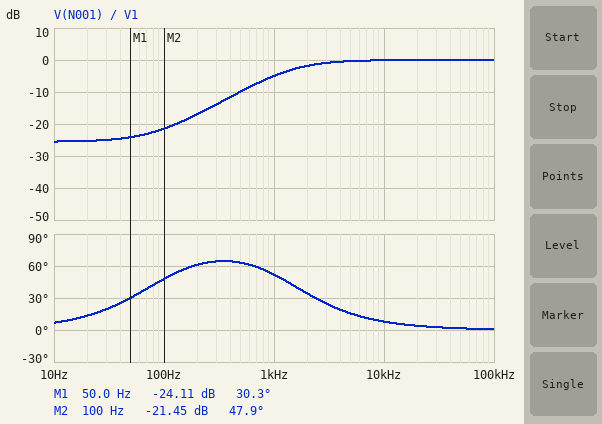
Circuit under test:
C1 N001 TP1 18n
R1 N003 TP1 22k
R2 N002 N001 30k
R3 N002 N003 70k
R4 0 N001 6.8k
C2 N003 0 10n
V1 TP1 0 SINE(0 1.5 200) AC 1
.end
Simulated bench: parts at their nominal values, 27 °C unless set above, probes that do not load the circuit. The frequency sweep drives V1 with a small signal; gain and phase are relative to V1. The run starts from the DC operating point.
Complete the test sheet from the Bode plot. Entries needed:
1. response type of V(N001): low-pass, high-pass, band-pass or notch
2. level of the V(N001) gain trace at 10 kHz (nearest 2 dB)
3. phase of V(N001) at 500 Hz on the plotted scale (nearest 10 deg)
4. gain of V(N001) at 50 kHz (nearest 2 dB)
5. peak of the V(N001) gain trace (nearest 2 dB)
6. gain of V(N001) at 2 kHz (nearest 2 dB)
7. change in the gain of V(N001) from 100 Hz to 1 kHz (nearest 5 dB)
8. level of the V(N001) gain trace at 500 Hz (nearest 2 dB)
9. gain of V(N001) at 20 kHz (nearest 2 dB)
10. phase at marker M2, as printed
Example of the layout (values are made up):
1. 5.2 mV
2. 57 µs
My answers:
1. high-pass
2. 0 dB
3. 60 deg
4. 0 dB
5. 0 dB
6. -2 dB
7. 15 dB
8. -10 dB
9. 0 dB
10. 47.9 deg
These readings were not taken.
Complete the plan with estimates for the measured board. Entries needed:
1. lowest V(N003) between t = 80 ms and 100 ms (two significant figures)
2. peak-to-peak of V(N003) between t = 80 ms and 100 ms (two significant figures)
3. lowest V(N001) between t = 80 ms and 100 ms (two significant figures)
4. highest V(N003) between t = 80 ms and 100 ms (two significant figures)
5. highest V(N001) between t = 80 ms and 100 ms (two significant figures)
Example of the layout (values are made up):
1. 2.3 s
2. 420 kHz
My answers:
1. -1.2 V
2. 2.4 V
3. -210 mV
4. 1.2 V
5. 210 mV
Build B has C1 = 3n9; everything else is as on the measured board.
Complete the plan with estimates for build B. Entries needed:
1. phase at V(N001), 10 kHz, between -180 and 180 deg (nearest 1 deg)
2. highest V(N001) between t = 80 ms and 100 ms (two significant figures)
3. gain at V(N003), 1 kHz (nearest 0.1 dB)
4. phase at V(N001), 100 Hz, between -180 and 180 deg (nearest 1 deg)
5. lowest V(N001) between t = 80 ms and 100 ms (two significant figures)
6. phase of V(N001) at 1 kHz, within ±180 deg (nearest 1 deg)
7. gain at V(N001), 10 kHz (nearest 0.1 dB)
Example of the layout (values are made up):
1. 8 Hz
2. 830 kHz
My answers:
1. 33 deg
2. 81 mV
3. -5.2 dB
4. 10 deg
5. -81 mV
6. 71 deg
7. -1.5 dB
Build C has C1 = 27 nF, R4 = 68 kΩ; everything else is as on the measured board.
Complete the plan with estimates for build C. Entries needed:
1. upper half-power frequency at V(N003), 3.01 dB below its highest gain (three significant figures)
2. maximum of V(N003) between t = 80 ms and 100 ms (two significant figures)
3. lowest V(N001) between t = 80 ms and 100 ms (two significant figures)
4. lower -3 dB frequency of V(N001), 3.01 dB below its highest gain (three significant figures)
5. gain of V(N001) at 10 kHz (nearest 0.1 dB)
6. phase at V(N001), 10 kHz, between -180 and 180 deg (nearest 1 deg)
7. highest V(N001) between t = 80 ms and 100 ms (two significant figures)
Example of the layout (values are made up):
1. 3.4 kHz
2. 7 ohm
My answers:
1. 991 Hz
2. 1.4 V
3. -1.2 V
4. 134 Hz
5. 0 dB
6. 1 deg
7. 1.2 V
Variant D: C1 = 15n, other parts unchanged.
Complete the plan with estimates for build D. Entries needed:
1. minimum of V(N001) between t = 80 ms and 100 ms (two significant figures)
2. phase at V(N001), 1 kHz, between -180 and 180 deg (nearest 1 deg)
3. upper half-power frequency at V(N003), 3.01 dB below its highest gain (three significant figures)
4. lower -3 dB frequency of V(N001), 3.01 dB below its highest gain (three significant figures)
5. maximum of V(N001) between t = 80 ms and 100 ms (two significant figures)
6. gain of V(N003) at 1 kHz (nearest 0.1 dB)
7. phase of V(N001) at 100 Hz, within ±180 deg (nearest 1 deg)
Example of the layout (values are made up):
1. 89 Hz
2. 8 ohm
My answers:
1. -180 mV
2. 56 deg
3. 967 Hz
4. 1.74 kHz
5. 180 mV
6. -4.8 dB
7. 43 deg
